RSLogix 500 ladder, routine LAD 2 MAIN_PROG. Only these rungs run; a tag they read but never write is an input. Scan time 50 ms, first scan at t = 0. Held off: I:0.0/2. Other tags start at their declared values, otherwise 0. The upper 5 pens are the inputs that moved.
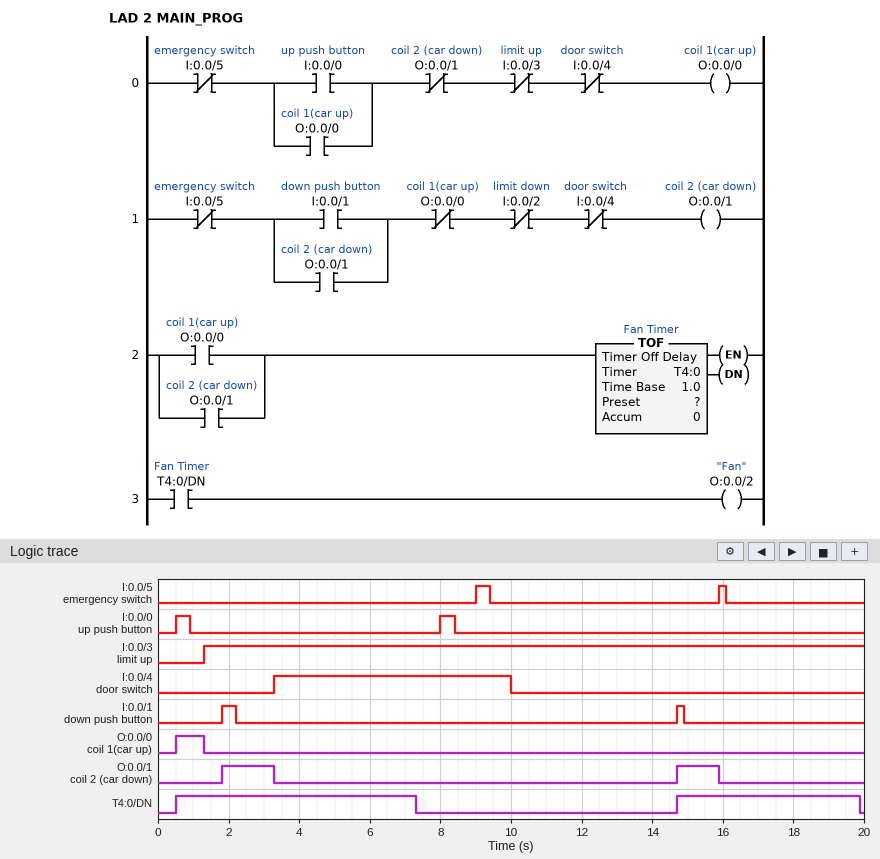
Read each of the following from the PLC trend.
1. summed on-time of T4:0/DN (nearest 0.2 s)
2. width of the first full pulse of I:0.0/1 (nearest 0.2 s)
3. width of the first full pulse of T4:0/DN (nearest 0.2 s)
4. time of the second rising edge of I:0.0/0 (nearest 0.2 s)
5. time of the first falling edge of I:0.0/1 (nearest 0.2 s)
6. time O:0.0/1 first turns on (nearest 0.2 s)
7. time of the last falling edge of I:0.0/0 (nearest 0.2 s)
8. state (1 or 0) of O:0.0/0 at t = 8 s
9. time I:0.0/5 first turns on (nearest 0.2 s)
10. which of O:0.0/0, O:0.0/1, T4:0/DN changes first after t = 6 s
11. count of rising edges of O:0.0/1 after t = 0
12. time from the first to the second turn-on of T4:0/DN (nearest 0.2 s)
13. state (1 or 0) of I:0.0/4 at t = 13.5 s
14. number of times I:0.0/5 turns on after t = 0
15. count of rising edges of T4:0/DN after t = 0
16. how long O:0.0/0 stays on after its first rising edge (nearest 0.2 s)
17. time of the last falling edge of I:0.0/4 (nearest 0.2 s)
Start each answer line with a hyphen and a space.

- 12.0 s
- 0.4 s
- 6.8 s
- 8.0 s
- 2.2 s
- 1.8 s
- 8.4 s
- 0
- 9.0 s
- T4:0/DN
- 2
- 14.2 s
- 0
- 2
- 2
- 0.8 s
- 10.0 s
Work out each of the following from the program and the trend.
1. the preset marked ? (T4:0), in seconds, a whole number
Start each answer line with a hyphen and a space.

- 4 s
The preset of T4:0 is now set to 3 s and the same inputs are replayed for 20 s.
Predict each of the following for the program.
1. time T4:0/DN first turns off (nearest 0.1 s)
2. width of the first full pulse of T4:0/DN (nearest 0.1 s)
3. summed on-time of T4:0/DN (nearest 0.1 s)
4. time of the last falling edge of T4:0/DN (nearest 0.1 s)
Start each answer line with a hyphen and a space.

- 6.3 s
- 5.8 s
- 10.0 s
- 18.9 s
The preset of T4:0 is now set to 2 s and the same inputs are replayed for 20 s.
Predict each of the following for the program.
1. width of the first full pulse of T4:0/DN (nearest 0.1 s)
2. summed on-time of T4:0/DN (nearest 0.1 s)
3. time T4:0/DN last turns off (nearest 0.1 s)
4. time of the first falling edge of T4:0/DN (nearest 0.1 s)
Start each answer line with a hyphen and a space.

- 4.8 s
- 8.0 s
- 17.9 s
- 5.3 s
